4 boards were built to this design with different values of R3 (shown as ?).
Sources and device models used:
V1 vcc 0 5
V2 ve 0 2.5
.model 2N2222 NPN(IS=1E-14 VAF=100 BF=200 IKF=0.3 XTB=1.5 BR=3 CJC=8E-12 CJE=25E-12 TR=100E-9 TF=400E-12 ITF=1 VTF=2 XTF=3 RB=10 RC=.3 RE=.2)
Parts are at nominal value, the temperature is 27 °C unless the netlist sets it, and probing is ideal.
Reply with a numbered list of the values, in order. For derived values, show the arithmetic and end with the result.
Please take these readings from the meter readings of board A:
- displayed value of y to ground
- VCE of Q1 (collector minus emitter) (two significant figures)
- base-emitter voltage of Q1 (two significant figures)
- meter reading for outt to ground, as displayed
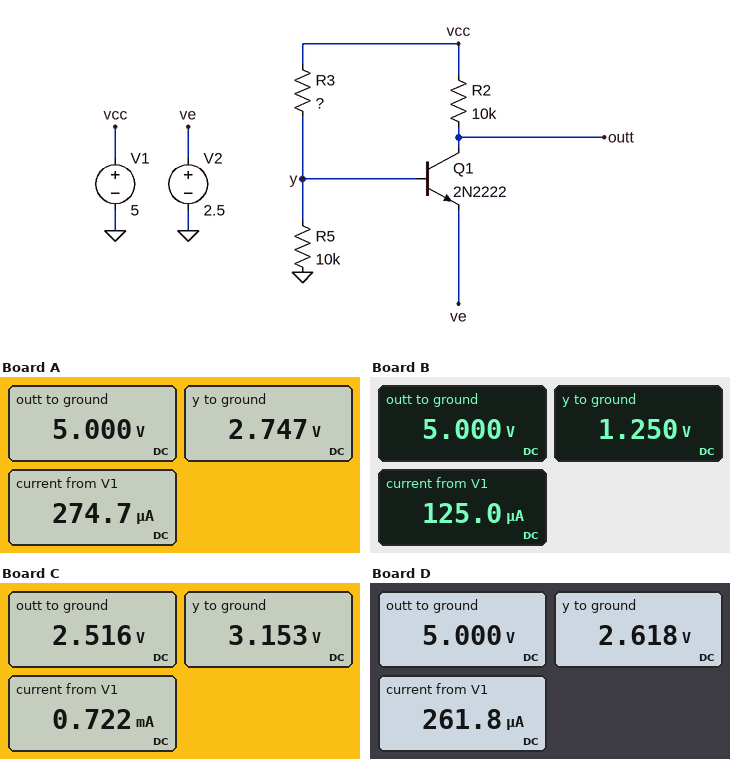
1. 2.747 V
2. 5 V - 2.5 V = 2.5 V
3. 2.747 V - 2.5 V = 250 mV
4. 5.000 V
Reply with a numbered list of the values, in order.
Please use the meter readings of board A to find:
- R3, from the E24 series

1. 8.2 kΩ
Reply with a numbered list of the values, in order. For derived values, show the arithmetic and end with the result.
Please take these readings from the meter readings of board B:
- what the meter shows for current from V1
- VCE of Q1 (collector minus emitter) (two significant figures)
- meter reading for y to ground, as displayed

1. 125.0 µA
2. 5 V - 2.5 V = 2.5 V
3. 1.250 V
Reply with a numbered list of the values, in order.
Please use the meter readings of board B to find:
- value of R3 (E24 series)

1. 30 kΩ
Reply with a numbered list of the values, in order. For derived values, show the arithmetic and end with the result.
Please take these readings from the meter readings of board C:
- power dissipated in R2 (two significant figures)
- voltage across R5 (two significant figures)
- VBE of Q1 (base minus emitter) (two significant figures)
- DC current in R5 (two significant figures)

1. (5 V - 2.516 V)^2 / 10 kΩ = 620 µW
2. 3.153 V = 3.2 V
3. 3.153 V - 2.5 V = 650 mV
4. (3.153 V) / 10 kΩ = 320 µA
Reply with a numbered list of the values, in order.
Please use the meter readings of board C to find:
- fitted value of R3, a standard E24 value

1. 3.9 kΩ
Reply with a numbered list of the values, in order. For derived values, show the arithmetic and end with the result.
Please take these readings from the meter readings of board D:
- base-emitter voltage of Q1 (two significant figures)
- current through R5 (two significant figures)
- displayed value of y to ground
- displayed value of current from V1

1. 2.618 V - 2.5 V = 120 mV
2. (2.618 V) / 10 kΩ = 260 µA
3. 2.618 V
4. 261.8 µA
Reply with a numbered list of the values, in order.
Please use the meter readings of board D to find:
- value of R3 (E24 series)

1. 9.1 kΩ
